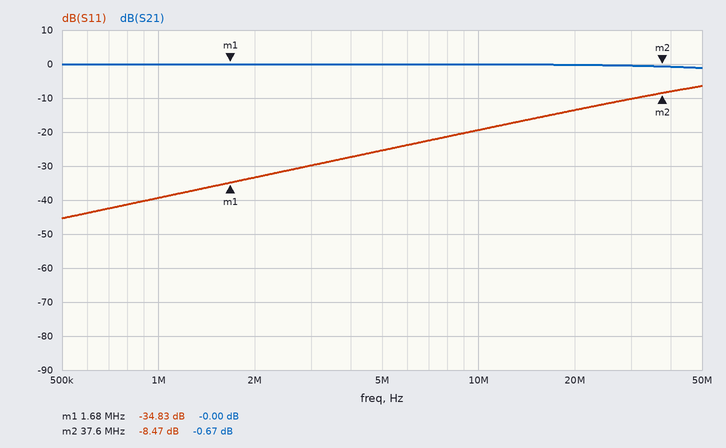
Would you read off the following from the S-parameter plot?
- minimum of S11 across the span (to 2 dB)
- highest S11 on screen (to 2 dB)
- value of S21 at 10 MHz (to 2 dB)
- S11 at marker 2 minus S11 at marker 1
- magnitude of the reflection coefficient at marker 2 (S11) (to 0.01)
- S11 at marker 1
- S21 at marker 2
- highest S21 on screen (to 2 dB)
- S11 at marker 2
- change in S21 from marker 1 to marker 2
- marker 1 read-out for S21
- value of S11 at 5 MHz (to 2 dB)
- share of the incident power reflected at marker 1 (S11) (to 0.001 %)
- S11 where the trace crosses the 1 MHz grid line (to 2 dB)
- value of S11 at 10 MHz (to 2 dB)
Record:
-46 dB
-6 dB
0 dB
26.36 dB
0.38
-34.83 dB
-0.67 dB
0 dB
-8.47 dB
-0.67 dB
-0.00 dB
-26 dB
0.033 %
-40 dB
-20 dB
